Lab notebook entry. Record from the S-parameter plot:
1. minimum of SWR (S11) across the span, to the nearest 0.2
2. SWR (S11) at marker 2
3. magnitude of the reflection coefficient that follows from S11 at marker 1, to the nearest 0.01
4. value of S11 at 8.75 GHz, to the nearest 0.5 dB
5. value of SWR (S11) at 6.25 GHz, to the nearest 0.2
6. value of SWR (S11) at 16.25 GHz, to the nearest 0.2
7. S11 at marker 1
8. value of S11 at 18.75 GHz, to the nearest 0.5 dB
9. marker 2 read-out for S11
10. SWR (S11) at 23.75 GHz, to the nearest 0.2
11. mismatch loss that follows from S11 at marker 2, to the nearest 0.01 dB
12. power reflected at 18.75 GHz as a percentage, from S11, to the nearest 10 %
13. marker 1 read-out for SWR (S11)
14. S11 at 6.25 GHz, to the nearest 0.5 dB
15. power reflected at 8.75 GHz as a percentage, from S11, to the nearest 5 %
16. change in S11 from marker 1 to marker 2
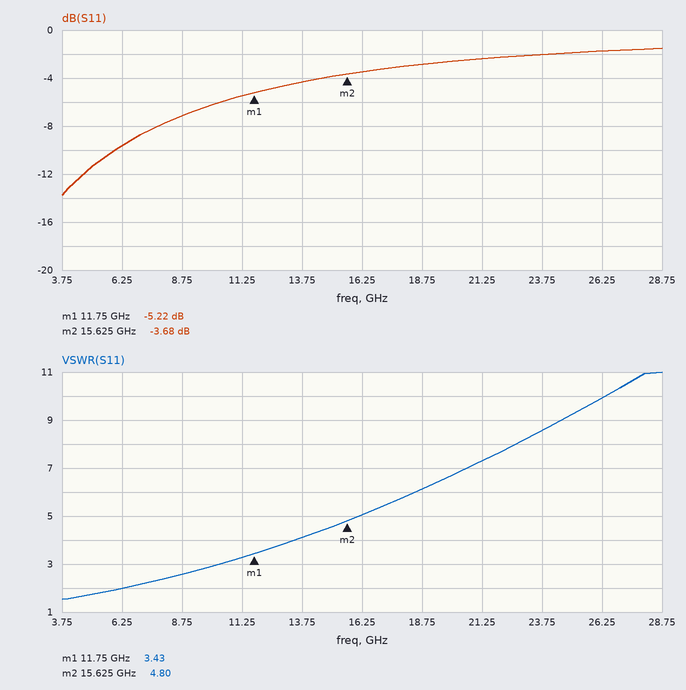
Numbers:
1.6
4.80
0.55
-7.0 dB
2.0
5.0
-5.22 dB
-3.0 dB
-3.68 dB
8.6
2.43 dB
50 %
3.43
-9.5 dB
20 %
1.54 dB
